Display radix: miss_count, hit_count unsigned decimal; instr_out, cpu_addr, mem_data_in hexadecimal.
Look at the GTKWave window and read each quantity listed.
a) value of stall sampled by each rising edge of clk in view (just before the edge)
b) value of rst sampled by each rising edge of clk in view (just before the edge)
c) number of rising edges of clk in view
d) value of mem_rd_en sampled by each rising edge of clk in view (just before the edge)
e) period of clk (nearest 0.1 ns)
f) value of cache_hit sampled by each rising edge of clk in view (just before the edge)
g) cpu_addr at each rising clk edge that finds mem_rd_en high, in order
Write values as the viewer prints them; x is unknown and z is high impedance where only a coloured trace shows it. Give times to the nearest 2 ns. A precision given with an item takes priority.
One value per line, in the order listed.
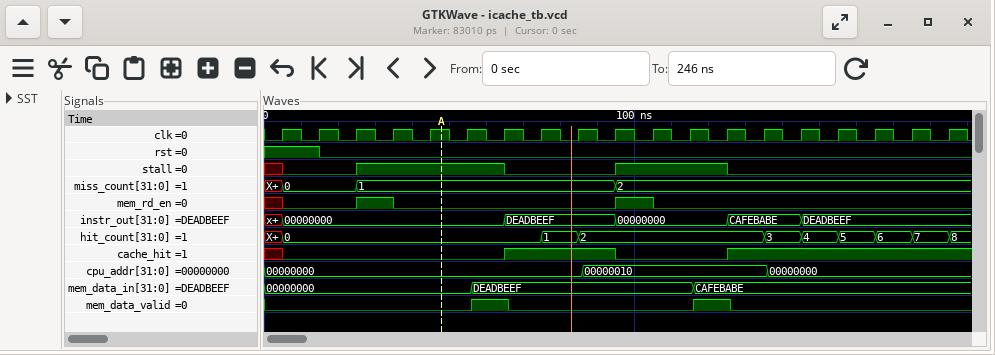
x 0 0 1 1 1 1 0 0 0 1 1 1 0 0 0 0 0 0
1 1 0 0 0 0 0 0 0 0 0 0 0 0 0 0 0 0 0
19
x 0 0 1 0 0 0 0 0 0 1 0 0 0 0 0 0 0 0
10 ns
x 0 0 0 0 0 0 1 1 1 0 0 0 1 1 1 1 1 1
00000000, 00000010
